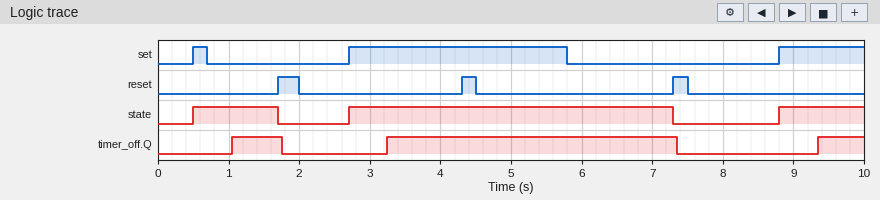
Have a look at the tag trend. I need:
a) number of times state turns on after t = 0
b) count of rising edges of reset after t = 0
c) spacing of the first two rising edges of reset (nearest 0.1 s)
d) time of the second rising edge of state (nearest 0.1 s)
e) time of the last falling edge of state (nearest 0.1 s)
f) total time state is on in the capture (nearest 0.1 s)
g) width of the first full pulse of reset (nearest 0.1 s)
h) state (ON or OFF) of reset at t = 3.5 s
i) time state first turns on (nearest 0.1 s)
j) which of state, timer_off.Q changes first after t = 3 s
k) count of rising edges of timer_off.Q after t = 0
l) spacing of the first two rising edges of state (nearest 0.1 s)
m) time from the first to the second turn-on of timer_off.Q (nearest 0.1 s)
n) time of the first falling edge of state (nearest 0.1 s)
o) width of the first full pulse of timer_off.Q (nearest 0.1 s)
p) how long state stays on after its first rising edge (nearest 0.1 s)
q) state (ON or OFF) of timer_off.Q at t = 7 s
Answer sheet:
3
3
2.6 s
2.7 s
7.3 s
7.0 s
0.3 s
OFF
0.5 s
timer_off.Q
3
2.2 s
2.2 s
1.7 s
0.7 s
1.2 s
ON
